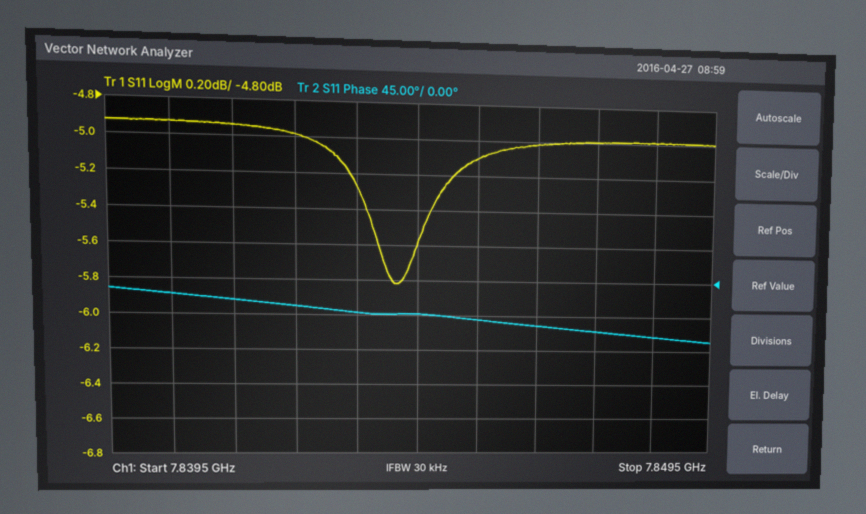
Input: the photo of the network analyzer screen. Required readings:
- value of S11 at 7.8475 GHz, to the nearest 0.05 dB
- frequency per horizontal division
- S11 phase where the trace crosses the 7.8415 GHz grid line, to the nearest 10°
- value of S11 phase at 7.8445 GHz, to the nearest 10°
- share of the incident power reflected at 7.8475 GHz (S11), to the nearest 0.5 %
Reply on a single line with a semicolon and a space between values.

-5.00 dB; 1 MHz; -30°; -40°; 31.5 %
